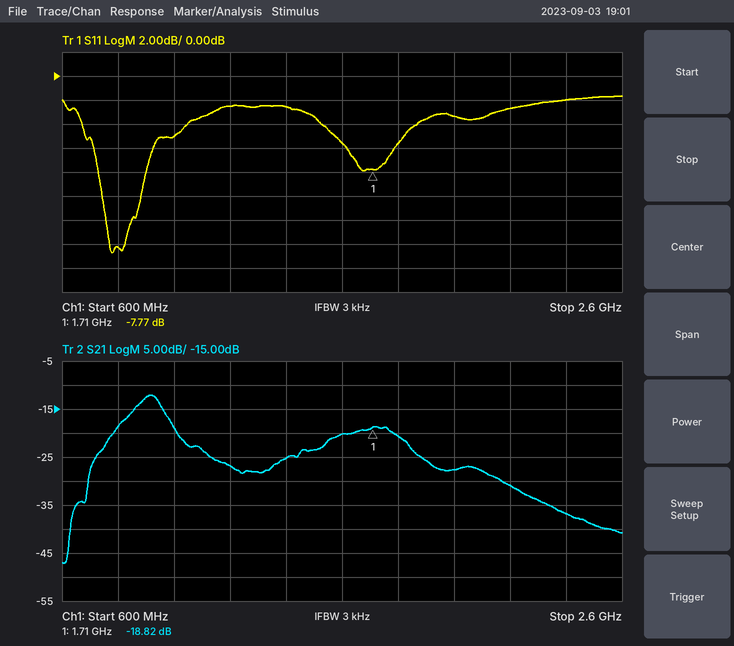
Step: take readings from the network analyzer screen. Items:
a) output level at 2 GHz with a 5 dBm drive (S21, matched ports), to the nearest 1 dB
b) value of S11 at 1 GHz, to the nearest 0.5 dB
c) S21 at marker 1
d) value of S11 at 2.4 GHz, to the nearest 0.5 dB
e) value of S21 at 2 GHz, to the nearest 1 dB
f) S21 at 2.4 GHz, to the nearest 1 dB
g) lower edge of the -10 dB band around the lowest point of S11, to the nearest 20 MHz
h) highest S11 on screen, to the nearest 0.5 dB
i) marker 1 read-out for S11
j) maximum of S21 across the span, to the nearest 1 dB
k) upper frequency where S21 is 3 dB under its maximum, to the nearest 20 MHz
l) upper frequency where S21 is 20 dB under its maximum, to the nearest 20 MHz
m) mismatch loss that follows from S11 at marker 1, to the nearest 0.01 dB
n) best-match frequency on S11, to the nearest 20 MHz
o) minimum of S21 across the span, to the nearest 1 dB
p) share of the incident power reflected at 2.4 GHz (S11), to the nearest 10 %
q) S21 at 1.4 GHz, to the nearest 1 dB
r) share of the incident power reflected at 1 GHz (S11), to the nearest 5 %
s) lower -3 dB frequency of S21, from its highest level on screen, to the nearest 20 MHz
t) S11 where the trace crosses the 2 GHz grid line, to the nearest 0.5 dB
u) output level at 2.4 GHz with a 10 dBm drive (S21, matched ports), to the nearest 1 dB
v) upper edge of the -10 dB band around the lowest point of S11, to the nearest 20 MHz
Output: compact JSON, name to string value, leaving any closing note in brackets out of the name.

{"output level at 2 GHz with a 5 dBm drive (S21, matched ports), to the nearest 1 dB": "-23 dBm", "value of S11 at 1 GHz, to the nearest 0.5 dB": "-5.0 dB", "S21 at marker 1": "-18.82 dB", "value of S11 at 2.4 GHz, to the nearest 0.5 dB": "-2.0 dB", "value of S21 at 2 GHz, to the nearest 1 dB": "-28 dB", "S21 at 2.4 GHz, to the nearest 1 dB": "-37 dB", "lower edge of the -10 dB band around the lowest point of S11, to the nearest 20 MHz": "740 MHz", "highest S11 on screen, to the nearest 0.5 dB": "-1.5 dB", "marker 1 read-out for S11": "-7.77 dB", "maximum of S21 across the span, to the nearest 1 dB": "-12 dB", "upper frequency where S21 is 3 dB under its maximum, to the nearest 20 MHz": "960 MHz", "upper frequency where S21 is 20 dB under its maximum, to the nearest 20 MHz": "2.24 GHz", "mismatch loss that follows from S11 at marker 1, to the nearest 0.01 dB": "0.79 dB", "best-match frequency on S11, to the nearest 20 MHz": "780 MHz", "minimum of S21 across the span, to the nearest 1 dB": "-47 dB", "share of the incident power reflected at 2.4 GHz (S11), to the nearest 10 %": "60 %", "S21 at 1.4 GHz, to the nearest 1 dB": "-25 dB", "share of the incident power reflected at 1 GHz (S11), to the nearest 5 %": "30 %", "lower -3 dB frequency of S21, from its highest level on screen, to the nearest 20 MHz": "860 MHz", "S11 where the trace crosses the 2 GHz grid line, to the nearest 0.5 dB": "-3.5 dB", "output level at 2.4 GHz with a 10 dBm drive (S21, matched ports), to the nearest 1 dB": "-27 dBm", "upper edge of the -10 dB band around the lowest point of S11, to the nearest 20 MHz": "880 MHz"}
